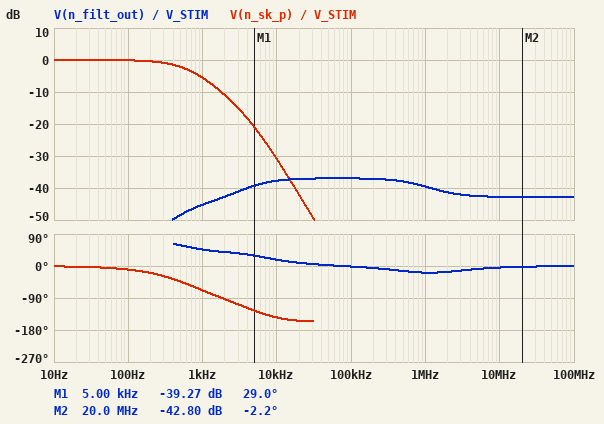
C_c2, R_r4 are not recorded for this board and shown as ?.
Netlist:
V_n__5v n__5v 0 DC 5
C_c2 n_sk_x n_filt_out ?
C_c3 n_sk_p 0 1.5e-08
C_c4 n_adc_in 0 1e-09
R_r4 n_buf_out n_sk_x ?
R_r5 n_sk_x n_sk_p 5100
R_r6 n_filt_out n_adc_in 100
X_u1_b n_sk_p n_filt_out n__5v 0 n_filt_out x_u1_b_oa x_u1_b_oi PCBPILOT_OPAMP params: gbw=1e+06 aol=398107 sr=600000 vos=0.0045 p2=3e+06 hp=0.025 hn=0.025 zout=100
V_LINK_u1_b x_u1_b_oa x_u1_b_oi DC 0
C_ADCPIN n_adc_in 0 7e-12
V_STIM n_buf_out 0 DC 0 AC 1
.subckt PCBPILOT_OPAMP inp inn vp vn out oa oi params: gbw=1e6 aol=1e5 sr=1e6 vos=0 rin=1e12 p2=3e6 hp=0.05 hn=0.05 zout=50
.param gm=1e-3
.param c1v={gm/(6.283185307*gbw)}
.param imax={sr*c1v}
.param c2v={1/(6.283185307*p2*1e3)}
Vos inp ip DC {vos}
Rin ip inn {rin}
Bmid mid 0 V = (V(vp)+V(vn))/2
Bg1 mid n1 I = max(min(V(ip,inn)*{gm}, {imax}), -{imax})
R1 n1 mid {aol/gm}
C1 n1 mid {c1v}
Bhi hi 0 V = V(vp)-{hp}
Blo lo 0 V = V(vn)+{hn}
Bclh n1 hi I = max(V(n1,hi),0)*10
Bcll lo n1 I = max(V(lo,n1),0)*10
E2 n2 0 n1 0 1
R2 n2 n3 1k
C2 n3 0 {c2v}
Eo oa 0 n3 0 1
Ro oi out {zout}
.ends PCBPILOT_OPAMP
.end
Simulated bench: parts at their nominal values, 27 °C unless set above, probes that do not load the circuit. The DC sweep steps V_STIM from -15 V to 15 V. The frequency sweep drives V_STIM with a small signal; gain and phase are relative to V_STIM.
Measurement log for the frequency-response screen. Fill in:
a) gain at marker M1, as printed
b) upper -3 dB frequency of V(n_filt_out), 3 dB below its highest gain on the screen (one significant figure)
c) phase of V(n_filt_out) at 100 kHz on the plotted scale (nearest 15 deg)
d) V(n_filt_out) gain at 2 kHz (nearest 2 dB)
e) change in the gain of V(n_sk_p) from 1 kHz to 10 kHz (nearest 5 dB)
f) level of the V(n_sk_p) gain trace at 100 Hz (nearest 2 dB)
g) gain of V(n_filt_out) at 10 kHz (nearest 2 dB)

-39.27 dB
1 MHz
0 deg
-42 dB
-25 dB
0 dB
-38 dB
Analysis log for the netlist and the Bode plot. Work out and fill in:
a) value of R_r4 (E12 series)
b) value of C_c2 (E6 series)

6.8 kΩ
15 nF
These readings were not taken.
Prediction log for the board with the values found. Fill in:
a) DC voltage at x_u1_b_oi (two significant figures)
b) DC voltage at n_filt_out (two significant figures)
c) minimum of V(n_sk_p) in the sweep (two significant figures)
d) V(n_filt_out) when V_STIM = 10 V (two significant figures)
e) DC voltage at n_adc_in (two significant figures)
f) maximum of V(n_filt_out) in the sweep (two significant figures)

25 mV
25 mV
-15 V
5.0 V
25 mV
5.0 V
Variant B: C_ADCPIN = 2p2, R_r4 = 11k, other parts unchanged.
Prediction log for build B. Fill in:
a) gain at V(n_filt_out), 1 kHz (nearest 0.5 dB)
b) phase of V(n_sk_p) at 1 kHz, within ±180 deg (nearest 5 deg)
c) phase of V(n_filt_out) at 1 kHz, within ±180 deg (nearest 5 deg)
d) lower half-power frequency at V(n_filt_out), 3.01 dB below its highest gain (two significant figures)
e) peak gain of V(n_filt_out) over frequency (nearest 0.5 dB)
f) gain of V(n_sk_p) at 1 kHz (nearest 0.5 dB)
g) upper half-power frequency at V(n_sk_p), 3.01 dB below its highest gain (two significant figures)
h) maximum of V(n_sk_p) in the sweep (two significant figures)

-48.0 dB
-80 deg
35 deg
3.5 kHz
-41.0 dB
-8.5 dB
420 Hz
15 V
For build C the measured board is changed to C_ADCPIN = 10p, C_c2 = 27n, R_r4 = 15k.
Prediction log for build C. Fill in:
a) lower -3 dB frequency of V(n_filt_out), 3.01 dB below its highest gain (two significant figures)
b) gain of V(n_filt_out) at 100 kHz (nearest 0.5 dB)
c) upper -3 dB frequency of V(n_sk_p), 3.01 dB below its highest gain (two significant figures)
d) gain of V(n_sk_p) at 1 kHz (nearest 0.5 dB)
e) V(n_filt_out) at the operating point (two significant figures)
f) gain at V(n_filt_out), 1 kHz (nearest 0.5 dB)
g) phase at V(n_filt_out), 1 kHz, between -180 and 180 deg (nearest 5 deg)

1.6 kHz
-44.0 dB
240 Hz
-13.0 dB
25 mV
-47.5 dB
20 deg
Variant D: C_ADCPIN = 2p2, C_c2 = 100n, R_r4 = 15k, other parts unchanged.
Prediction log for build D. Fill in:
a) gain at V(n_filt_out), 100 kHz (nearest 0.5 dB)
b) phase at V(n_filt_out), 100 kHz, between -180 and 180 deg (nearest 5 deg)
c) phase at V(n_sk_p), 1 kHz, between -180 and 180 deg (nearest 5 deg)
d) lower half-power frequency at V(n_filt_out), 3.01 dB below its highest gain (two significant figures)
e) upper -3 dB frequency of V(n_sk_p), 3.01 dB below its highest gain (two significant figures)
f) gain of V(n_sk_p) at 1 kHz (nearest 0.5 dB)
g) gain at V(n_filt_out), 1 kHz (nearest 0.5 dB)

-44.0 dB
-5 deg
-105 deg
120 Hz
91 Hz
-21.5 dB
-44.5 dB
